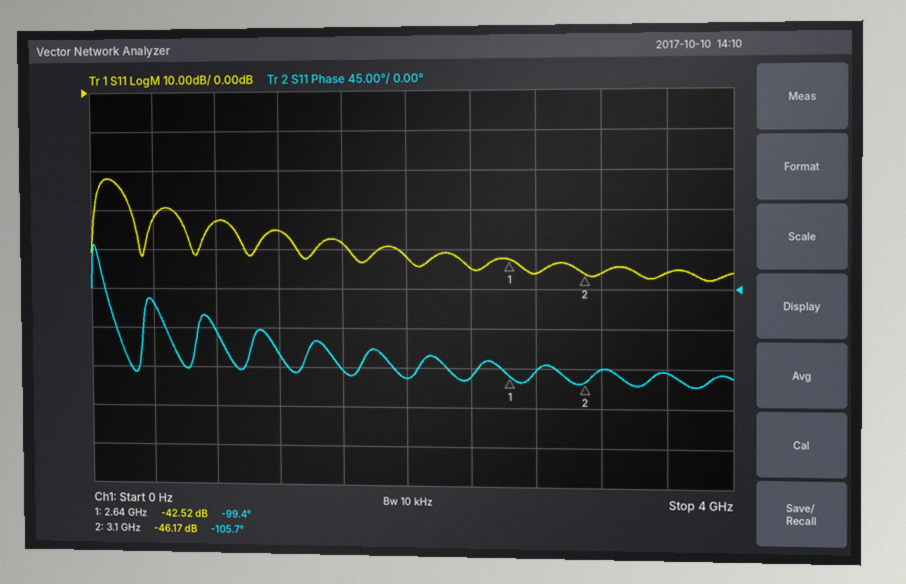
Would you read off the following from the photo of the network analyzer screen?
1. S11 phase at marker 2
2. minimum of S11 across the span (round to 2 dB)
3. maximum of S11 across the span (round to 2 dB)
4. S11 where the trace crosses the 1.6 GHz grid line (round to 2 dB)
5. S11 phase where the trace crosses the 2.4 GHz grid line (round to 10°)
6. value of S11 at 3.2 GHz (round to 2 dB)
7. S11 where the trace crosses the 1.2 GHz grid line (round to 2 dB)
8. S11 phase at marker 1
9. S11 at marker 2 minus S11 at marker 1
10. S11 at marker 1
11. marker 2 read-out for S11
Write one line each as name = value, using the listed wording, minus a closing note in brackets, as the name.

S11 phase at marker 2 = -105.7°
minimum of S11 across the span = -48 dB
maximum of S11 across the span = -22 dB
S11 where the trace crosses the 1.6 GHz grid line = -38 dB
S11 phase where the trace crosses the 2.4 GHz grid line = -100°
value of S11 at 3.2 GHz = -46 dB
S11 where the trace crosses the 1.2 GHz grid line = -36 dB
S11 phase at marker 1 = -99.4°
S11 at marker 2 minus S11 at marker 1 = -3.65 dB
S11 at marker 1 = -42.52 dB
marker 2 read-out for S11 = -46.17 dB
